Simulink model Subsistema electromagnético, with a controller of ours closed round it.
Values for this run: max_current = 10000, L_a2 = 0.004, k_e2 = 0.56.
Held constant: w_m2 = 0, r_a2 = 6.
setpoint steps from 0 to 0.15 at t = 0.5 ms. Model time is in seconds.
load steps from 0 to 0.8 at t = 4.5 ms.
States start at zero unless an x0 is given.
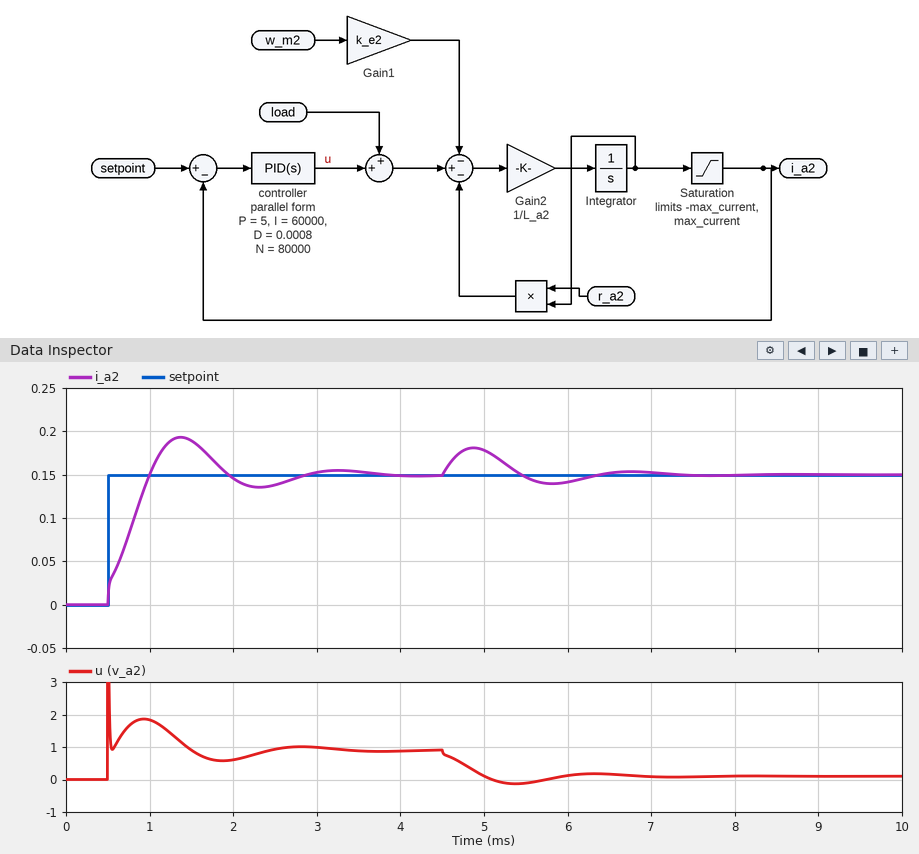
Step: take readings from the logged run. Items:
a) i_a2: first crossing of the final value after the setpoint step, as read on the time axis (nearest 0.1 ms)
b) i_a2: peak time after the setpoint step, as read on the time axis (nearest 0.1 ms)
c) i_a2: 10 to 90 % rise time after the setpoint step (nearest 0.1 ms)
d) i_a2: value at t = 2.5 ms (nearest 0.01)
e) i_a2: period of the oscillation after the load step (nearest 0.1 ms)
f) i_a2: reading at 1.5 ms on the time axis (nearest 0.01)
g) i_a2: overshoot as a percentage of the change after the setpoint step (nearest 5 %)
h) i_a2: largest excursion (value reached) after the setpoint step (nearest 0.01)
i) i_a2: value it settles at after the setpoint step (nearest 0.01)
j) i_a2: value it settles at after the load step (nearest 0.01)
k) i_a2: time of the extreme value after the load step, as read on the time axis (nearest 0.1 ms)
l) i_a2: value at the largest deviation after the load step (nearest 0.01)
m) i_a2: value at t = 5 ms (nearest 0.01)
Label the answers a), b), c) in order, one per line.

a) 1.0 ms
b) 1.4 ms
c) 0.4 ms
d) 0.14
e) 1.9 ms
f) 0.19
g) 30 %
h) 0.19
i) 0.15
j) 0.15
k) 4.9 ms
l) 0.18
m) 0.18
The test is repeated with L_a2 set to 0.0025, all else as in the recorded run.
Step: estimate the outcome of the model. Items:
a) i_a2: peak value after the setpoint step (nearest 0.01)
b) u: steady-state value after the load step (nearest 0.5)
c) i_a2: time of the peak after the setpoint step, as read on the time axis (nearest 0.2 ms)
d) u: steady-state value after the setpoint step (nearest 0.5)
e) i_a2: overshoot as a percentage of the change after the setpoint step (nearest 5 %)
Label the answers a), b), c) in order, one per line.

a) 0.18
b) 0.0
c) 1.2 ms
d) 1.0
e) 20 %
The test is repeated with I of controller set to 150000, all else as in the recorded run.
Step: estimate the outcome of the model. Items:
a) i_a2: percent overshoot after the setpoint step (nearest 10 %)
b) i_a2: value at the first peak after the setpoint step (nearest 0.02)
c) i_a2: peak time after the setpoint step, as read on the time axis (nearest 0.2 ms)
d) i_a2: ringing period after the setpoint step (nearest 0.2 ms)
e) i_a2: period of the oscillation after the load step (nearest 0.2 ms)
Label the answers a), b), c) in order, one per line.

a) 40 %
b) 0.22
c) 1.0 ms
d) 1.2 ms
e) 1.2 ms
